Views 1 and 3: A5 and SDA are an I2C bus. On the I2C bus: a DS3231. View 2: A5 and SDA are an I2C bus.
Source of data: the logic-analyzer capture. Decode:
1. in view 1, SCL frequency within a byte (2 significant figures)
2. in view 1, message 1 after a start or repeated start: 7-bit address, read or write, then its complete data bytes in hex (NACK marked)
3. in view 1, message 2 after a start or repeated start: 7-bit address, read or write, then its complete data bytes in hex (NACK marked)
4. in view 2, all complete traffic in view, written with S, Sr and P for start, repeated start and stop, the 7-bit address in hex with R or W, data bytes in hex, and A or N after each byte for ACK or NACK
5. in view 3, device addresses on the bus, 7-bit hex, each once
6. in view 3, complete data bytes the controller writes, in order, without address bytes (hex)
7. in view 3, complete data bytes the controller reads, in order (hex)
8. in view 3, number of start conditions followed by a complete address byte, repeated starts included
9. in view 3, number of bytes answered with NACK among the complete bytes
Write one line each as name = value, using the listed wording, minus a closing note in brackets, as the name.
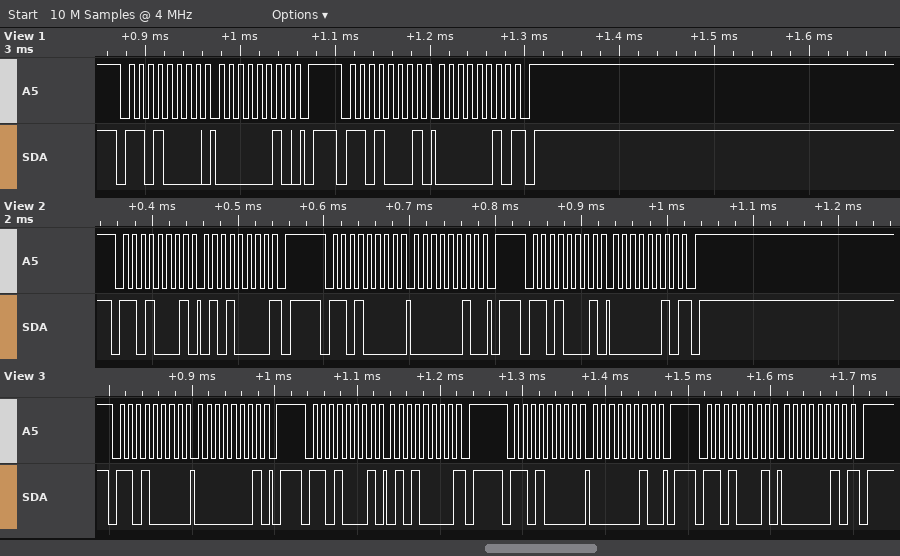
in view 1, SCL frequency within a byte = 100 kHz
in view 1, message 1 after a start or repeated start: 7-bit address, read or write, then its complete data bytes in hex = 0x68 write: 02
in view 1, message 2 after a start or repeated start: 7-bit address, read or write, then its complete data bytes in hex = 0x68 read: 02 NACK
in view 2, all complete traffic in view, written with S, Sr and P for start, repeated start and stop, the 7-bit address in hex with R or W, data bytes in hex, and A or N after each byte for ACK or NACK = S 68R A 50 N P S 68W A 02 A P S 68R A 02 N P
in view 3, device addresses on the bus, 7-bit hex, each once = 0x68
in view 3, complete data bytes the controller writes, in order, without address bytes = 01 02
in view 3, complete data bytes the controller reads, in order = 50 02
in view 3, number of start conditions followed by a complete address byte, repeated starts included = 4
in view 3, number of bytes answered with NACK among the complete bytes = 2
